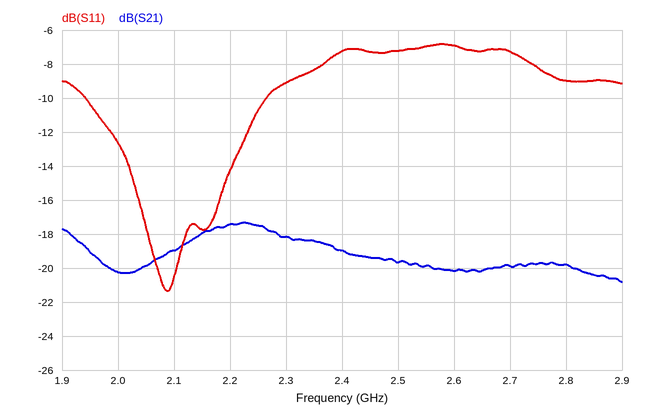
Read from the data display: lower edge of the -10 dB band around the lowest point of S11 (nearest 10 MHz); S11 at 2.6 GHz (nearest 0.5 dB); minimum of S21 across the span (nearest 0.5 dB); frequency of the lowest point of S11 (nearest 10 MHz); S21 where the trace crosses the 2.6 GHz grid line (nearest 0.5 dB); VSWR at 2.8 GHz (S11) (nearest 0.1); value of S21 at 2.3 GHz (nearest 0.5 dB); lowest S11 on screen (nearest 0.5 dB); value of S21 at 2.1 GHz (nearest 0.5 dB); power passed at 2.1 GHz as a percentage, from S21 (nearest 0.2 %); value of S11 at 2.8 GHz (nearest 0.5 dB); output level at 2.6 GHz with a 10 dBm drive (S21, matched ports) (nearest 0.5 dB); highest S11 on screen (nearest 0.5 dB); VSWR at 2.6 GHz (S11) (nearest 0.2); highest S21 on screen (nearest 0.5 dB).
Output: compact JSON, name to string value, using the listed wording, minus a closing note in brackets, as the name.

{"lower edge of the -10 dB band around the lowest point of S11": "1.94 GHz", "S11 at 2.6 GHz": "-7.0 dB", "minimum of S21 across the span": "-21.0 dB", "frequency of the lowest point of S11": "2.09 GHz", "S21 where the trace crosses the 2.6 GHz grid line": "-20.0 dB", "VSWR at 2.8 GHz (S11)": "2.1", "value of S21 at 2.3 GHz": "-18.0 dB", "lowest S11 on screen": "-21.5 dB", "value of S21 at 2.1 GHz": "-19.0 dB", "power passed at 2.1 GHz as a percentage, from S21": "1.2 %", "value of S11 at 2.8 GHz": "-9.0 dB", "output level at 2.6 GHz with a 10 dBm drive (S21, matched ports)": "-10.0 dBm", "highest S11 on screen": "-7.0 dB", "VSWR at 2.6 GHz (S11)": "2.6", "highest S21 on screen": "-17.5 dB"}
